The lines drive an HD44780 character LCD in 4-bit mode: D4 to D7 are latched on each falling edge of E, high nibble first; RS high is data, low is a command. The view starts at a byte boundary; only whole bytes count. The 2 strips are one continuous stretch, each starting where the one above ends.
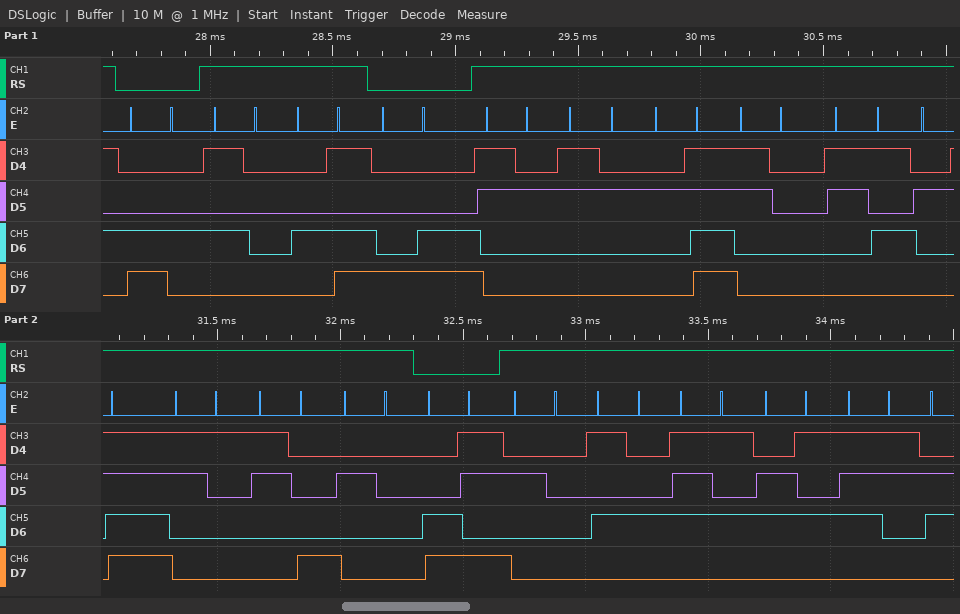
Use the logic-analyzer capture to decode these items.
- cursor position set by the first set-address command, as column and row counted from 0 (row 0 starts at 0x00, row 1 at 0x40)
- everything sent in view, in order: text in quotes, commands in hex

column 4, row 1
0xC4 "PM" 0x8C "22/05/18 " 0xCB " Tues"
